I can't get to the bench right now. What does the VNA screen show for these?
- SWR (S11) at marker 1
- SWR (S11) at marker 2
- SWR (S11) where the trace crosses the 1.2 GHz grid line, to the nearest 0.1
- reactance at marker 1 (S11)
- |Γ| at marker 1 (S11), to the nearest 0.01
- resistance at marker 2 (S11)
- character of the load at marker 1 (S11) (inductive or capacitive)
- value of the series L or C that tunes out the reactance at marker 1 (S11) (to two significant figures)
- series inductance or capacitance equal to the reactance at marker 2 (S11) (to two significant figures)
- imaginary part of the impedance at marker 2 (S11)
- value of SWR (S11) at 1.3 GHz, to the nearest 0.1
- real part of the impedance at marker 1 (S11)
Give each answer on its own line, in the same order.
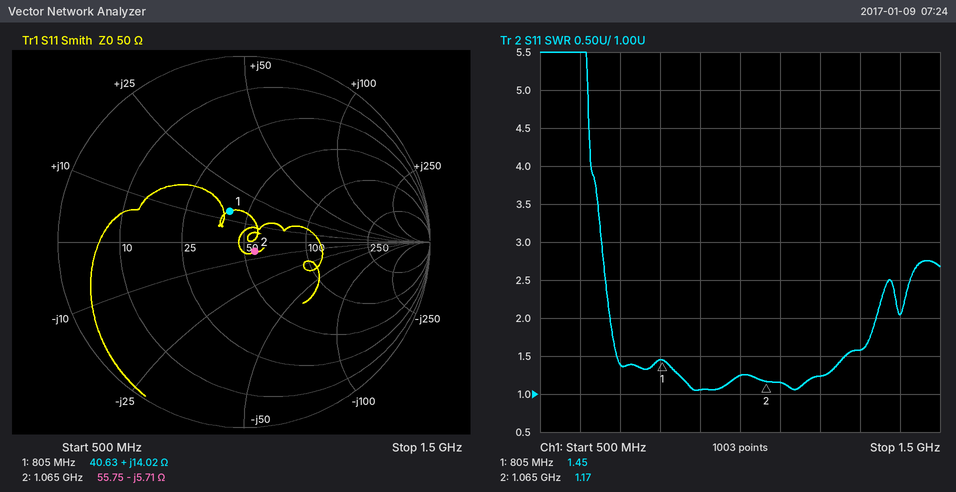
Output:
1.45
1.17
1.2
+14.02 Ω
0.18
55.75 Ω
inductive
14 pF
26 pF
-5.71 Ω
1.6
40.63 Ω
